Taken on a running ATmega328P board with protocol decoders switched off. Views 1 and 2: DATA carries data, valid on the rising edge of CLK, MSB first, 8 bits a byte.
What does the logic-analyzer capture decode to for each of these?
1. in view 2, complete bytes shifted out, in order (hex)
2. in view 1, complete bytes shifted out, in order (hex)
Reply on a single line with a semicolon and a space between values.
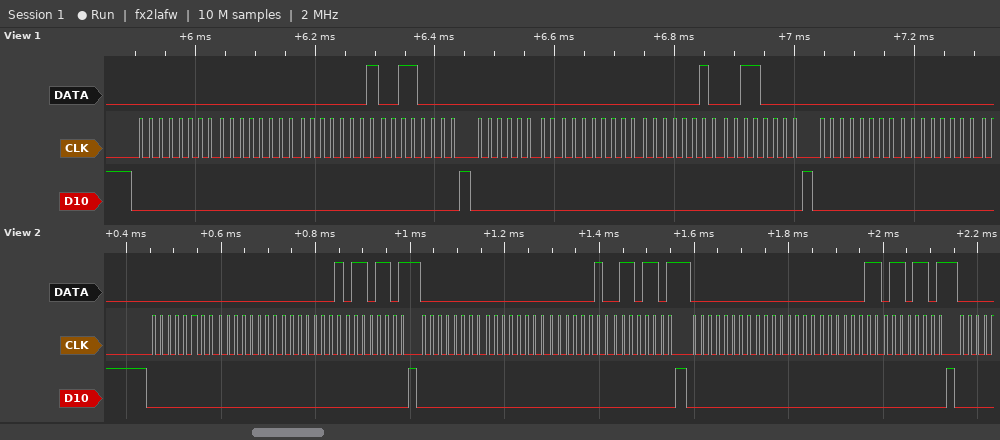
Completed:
00 00 01 6D 00 00 02 6D 00 00 03 6D; 0x00 0x00 0x01 0x30 0x00 0x00 0x02 0x30 0x00 0x00
